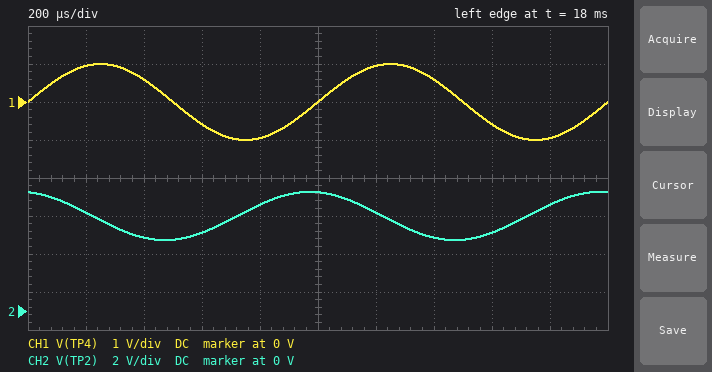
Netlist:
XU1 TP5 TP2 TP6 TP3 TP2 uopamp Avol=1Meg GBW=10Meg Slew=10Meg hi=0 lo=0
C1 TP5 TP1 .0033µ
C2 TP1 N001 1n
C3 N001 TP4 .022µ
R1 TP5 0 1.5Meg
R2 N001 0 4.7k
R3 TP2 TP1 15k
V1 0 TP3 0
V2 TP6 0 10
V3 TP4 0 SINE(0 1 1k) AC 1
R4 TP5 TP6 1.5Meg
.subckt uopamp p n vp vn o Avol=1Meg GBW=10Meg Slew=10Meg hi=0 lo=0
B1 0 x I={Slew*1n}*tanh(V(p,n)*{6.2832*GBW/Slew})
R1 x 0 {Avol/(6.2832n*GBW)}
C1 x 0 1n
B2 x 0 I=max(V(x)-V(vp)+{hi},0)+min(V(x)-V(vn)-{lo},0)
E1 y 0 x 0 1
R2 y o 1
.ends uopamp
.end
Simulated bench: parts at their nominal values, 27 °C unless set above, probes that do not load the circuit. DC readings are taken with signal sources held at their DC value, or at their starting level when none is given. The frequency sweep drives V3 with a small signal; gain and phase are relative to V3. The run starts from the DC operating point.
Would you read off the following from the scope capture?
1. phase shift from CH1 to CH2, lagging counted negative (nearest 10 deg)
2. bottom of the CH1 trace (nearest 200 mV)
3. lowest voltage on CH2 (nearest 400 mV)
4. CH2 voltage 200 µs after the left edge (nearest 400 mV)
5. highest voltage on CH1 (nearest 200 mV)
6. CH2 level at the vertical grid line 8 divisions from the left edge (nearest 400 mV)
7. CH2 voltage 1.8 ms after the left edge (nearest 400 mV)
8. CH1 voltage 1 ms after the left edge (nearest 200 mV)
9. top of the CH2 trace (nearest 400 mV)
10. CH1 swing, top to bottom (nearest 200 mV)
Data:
100 deg
-1.0 V
3.6 V
5.2 V
1.0 V
4.0 V
5.6 V
0 V
6.4 V
2.0 V
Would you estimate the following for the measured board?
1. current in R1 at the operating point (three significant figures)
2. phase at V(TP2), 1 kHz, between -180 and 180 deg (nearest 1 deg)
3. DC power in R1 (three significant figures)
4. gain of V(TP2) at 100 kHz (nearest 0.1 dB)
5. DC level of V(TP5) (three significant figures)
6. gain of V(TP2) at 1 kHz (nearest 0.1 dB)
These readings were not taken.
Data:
3.33 µA
100 deg
16.7 µW
0 dB
5.00 V
2.1 dB
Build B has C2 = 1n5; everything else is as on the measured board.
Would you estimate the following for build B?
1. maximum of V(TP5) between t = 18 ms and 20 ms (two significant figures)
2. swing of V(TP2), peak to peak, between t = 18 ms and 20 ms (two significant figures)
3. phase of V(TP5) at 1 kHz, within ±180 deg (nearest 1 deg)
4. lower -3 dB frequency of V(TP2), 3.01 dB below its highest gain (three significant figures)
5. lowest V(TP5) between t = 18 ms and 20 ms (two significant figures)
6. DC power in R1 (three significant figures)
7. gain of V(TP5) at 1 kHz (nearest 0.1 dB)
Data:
5.9 V
1.9 V
79 deg
618 Hz
4.1 V
16.7 µW
-0.6 dB
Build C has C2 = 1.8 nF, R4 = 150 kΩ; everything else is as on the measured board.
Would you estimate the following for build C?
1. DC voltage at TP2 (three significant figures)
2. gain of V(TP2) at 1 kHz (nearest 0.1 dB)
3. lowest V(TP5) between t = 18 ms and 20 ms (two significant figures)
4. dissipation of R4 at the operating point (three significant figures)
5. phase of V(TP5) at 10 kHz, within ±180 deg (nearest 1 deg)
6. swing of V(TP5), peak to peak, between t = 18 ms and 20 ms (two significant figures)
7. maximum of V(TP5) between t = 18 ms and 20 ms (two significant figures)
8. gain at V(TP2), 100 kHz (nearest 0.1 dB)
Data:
9.09 V
-9.1 dB
8.7 V
5.51 µW
15 deg
700 mV
9.4 V
0 dB
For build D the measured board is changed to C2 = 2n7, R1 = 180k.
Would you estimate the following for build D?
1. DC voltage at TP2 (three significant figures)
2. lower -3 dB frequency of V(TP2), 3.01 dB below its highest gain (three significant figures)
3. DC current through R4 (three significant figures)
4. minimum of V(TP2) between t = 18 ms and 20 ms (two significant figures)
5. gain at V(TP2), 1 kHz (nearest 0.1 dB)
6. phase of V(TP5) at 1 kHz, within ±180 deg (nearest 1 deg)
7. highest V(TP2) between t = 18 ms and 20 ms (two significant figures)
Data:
1.07 V
1.02 kHz
5.95 µA
370 mV
-3.0 dB
162 deg
1.8 V
